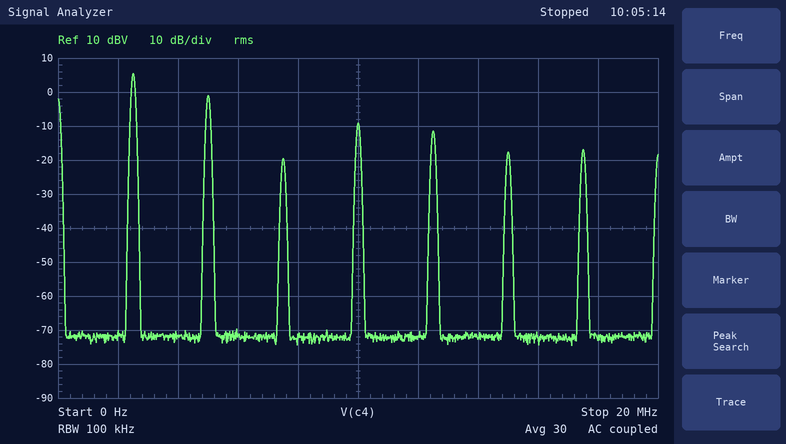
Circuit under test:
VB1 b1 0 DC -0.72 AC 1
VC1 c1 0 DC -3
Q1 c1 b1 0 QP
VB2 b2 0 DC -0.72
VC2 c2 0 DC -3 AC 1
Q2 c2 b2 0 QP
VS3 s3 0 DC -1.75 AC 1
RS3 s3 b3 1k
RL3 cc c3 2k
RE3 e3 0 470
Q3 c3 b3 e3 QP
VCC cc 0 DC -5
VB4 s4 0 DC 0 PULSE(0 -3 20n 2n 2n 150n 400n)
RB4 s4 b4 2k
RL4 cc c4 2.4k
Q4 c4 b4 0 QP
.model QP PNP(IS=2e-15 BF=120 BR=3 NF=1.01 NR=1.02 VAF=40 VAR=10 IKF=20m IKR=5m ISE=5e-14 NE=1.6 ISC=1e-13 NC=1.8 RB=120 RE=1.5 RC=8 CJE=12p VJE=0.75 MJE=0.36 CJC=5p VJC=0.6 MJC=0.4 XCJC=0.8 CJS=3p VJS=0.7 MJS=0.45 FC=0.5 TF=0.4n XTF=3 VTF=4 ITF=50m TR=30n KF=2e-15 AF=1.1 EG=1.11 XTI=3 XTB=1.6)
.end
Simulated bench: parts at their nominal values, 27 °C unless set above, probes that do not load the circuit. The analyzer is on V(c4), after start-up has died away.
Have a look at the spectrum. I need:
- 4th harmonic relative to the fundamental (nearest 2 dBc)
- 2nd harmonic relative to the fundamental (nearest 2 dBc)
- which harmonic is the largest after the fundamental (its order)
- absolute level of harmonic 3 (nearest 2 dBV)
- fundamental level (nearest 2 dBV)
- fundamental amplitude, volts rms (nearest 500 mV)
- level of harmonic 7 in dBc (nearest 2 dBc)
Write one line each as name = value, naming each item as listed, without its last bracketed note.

4th harmonic relative to the fundamental = -14 dBc
2nd harmonic relative to the fundamental = -6 dBc
which harmonic is the largest after the fundamental = 2
absolute level of harmonic 3 = -20 dBV
fundamental level = 6 dBV
fundamental amplitude, volts rms = 2.0 V
level of harmonic 7 in dBc = -22 dBc
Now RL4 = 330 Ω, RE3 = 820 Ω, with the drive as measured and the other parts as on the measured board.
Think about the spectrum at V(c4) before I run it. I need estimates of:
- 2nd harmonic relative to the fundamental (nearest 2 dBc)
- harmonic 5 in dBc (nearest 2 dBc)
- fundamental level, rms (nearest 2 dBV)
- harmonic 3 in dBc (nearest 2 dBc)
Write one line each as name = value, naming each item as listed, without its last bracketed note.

2nd harmonic relative to the fundamental = -20 dBc
harmonic 5 in dBc = -20 dBc
fundamental level, rms = 6 dBV
harmonic 3 in dBc = -12 dBc
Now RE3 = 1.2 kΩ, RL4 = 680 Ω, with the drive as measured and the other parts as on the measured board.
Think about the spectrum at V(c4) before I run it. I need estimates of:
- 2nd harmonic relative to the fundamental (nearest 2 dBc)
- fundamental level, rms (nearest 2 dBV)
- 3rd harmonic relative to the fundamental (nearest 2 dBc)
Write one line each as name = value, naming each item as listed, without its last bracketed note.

2nd harmonic relative to the fundamental = -10 dBc
fundamental level, rms = 6 dBV
3rd harmonic relative to the fundamental = -16 dBc
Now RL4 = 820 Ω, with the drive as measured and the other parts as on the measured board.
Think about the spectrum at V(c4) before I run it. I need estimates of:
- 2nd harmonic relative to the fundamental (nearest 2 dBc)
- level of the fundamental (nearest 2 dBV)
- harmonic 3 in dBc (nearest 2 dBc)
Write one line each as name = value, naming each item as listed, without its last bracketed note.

2nd harmonic relative to the fundamental = -10 dBc
level of the fundamental = 6 dBV
harmonic 3 in dBc = -18 dBc
